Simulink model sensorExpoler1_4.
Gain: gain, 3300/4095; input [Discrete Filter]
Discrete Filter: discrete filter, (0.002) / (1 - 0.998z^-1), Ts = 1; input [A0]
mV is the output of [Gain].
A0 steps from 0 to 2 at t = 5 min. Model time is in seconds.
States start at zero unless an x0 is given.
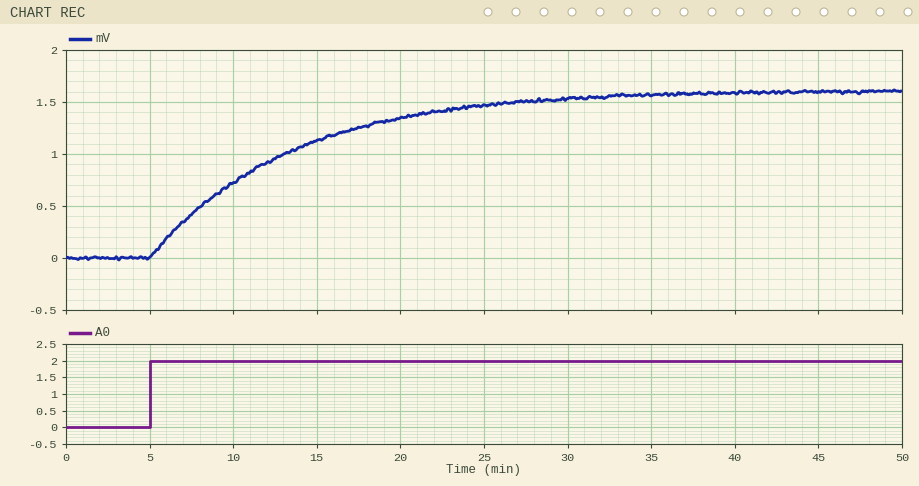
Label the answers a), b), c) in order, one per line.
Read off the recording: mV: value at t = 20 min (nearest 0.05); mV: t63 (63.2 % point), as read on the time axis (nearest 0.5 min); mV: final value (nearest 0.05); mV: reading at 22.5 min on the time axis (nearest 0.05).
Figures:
a) 1.35
b) 13.5 min
c) 1.60
d) 1.40
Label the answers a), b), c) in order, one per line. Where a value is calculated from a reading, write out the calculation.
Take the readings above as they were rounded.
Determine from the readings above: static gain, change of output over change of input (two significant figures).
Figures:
a) (1.6 - 0) / (2 - 0) = 0.80
